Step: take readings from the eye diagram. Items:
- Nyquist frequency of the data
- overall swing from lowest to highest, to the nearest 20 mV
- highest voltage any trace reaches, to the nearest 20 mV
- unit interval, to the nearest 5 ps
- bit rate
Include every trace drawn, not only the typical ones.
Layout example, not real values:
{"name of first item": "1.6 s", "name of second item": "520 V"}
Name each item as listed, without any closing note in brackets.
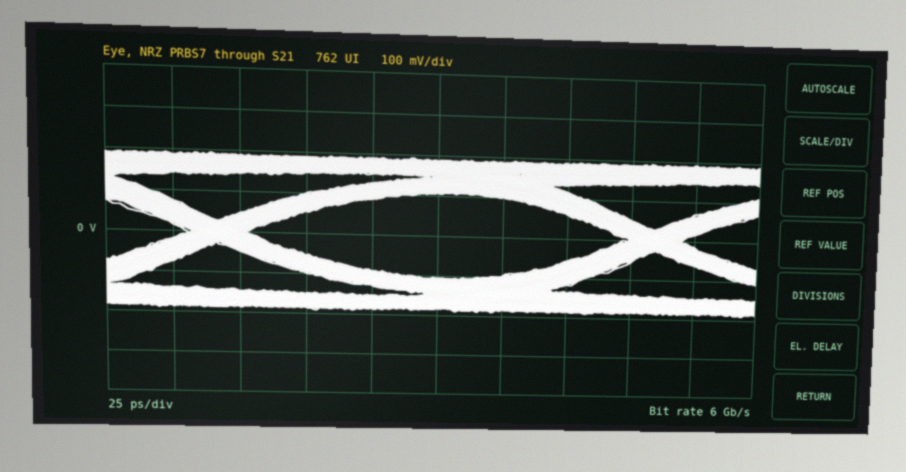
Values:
{"Nyquist frequency of the data": "3 GHz", "overall swing from lowest to highest, to the nearest 20 mV": "380 mV", "highest voltage any trace reaches, to the nearest 20 mV": "200 mV", "unit interval, to the nearest 5 ps": "165 ps", "bit rate": "6 Gb/s"}
